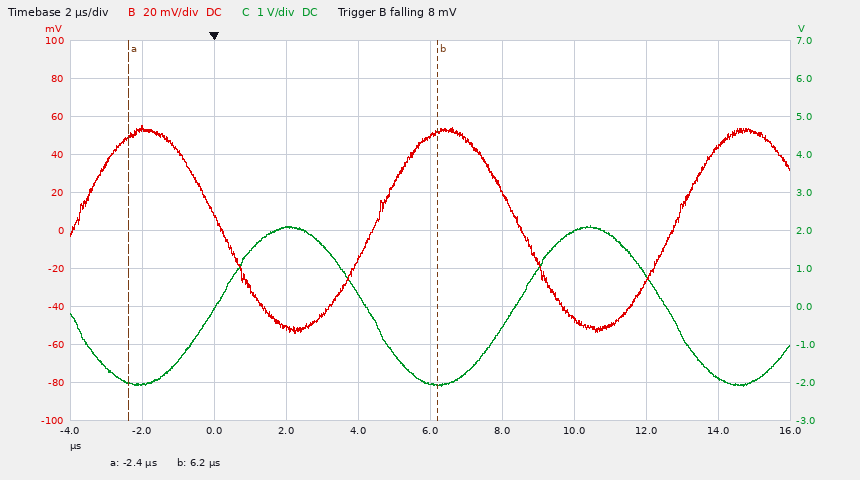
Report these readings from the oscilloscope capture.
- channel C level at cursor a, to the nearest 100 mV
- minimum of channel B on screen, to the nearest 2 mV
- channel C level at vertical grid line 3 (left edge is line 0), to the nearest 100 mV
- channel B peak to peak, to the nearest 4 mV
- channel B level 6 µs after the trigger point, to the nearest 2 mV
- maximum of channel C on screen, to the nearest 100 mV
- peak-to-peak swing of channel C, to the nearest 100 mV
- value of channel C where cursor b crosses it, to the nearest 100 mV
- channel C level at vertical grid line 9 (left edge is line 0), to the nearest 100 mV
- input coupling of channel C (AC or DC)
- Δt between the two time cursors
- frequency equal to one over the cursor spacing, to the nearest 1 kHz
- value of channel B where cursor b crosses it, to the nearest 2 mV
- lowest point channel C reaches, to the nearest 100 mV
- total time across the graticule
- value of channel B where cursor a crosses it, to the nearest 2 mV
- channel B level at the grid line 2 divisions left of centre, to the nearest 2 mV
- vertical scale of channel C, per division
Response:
-2.0 V
-54 mV
2.1 V
108 mV
50 mV
2.1 V
4.2 V
-2.1 V
-1.9 V
DC
8.6 µs
116 kHz
52 mV
-2.1 V
20 µs
50 mV
-52 mV
1 V
